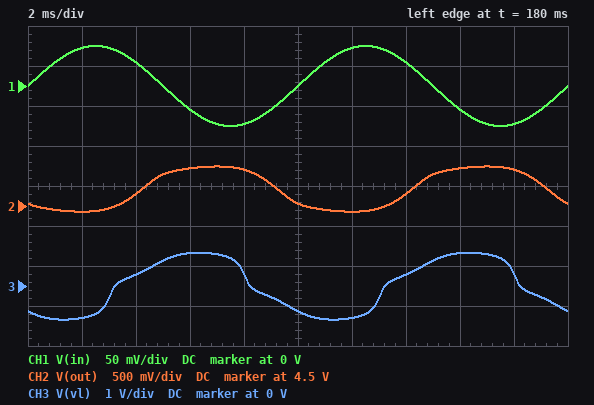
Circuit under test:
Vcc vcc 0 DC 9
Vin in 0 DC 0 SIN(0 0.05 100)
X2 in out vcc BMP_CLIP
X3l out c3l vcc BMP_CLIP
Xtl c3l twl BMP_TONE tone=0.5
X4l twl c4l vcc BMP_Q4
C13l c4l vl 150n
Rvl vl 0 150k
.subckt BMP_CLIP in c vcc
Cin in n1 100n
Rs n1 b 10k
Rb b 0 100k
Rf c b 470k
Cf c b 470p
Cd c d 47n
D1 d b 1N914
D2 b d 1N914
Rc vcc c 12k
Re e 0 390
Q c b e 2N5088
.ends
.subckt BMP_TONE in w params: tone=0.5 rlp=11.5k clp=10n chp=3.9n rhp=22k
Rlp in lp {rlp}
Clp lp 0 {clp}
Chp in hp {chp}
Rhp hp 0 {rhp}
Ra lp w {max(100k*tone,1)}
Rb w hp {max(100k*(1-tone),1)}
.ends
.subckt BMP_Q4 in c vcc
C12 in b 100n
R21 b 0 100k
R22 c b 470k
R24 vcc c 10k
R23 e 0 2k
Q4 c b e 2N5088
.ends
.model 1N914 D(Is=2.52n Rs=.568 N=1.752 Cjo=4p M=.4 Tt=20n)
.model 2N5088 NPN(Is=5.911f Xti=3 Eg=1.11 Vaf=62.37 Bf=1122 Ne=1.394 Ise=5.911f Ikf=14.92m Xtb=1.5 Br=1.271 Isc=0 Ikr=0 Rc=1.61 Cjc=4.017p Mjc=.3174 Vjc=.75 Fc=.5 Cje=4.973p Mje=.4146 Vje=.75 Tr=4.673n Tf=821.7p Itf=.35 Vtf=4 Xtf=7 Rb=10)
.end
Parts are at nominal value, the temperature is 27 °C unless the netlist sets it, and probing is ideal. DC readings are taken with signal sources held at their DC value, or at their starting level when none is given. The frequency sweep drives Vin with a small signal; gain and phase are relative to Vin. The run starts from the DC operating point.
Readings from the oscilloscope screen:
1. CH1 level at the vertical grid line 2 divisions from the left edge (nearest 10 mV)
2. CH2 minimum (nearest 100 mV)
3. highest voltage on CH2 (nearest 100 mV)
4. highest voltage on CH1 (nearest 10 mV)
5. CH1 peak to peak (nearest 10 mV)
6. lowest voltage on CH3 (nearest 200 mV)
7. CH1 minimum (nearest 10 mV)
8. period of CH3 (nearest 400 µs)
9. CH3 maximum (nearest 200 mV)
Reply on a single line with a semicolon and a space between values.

30 mV; 4.4 V; 5.0 V; 50 mV; 100 mV; -800 mV; -50 mV; 10.0 ms; 800 mV
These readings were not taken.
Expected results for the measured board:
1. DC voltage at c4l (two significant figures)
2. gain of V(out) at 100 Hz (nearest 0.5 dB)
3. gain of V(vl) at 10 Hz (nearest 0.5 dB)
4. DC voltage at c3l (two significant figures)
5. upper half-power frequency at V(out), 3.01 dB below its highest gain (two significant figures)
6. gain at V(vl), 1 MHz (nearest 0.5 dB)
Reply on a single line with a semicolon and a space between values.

6.5 V; 20.0 dB; 7.0 dB; 4.6 V; 2.3 kHz; -53.5 dB
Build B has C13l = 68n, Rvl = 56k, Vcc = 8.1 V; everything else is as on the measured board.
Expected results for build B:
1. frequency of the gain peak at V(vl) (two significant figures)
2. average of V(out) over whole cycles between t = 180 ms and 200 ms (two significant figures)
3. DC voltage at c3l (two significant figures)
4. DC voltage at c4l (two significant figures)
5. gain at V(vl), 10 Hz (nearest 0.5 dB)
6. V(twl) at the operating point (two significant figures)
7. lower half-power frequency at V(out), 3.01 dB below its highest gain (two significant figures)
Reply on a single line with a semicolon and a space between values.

240 Hz; 4.5 V; 4.4 V; 6.0 V; -4.0 dB; 2.4 V; 41 Hz
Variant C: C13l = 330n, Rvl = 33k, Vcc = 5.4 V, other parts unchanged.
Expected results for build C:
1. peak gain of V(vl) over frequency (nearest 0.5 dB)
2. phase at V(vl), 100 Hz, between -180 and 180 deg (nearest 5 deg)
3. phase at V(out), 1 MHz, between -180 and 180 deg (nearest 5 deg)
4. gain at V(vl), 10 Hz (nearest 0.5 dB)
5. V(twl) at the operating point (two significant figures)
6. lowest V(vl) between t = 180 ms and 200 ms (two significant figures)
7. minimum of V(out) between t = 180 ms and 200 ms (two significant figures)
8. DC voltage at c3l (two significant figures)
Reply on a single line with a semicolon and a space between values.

39.0 dB; -120 deg; 30 deg; 2.0 dB; 2.0 V; -590 mV; 3.6 V; 3.8 V
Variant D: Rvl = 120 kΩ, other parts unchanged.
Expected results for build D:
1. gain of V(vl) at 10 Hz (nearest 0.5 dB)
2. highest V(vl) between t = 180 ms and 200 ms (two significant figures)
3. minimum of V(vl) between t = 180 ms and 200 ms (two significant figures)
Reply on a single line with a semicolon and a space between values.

6.5 dB; 820 mV; -830 mV
